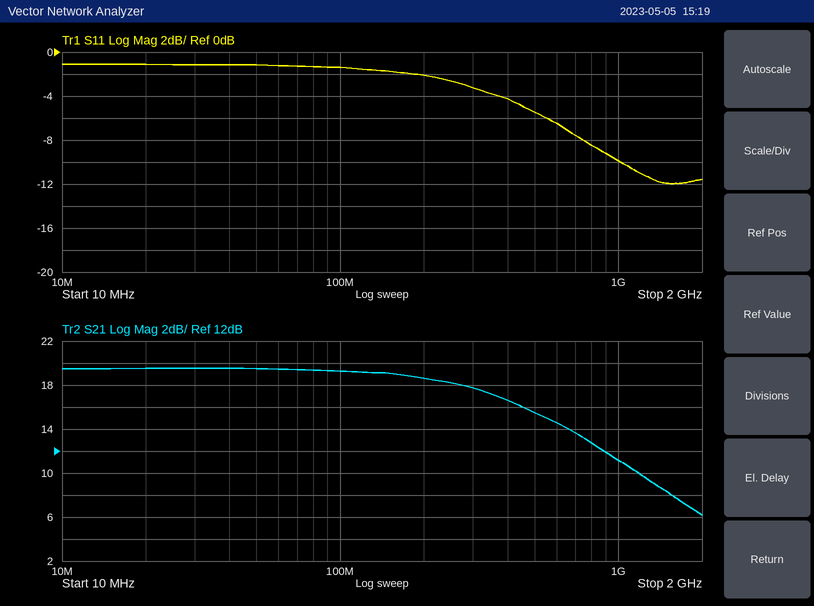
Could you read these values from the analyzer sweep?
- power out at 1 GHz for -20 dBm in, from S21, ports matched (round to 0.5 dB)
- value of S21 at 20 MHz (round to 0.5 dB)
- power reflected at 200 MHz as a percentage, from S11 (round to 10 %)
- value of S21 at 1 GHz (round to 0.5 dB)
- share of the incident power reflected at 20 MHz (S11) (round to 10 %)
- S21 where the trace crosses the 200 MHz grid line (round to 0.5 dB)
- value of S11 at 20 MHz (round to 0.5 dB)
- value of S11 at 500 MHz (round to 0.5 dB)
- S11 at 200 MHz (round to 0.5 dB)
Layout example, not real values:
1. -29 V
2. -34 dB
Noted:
1. -9.0 dBm
2. 19.5 dB
3. 60 %
4. 11.0 dB
5. 80 %
6. 18.5 dB
7. -1.0 dB
8. -5.5 dB
9. -2.0 dB
